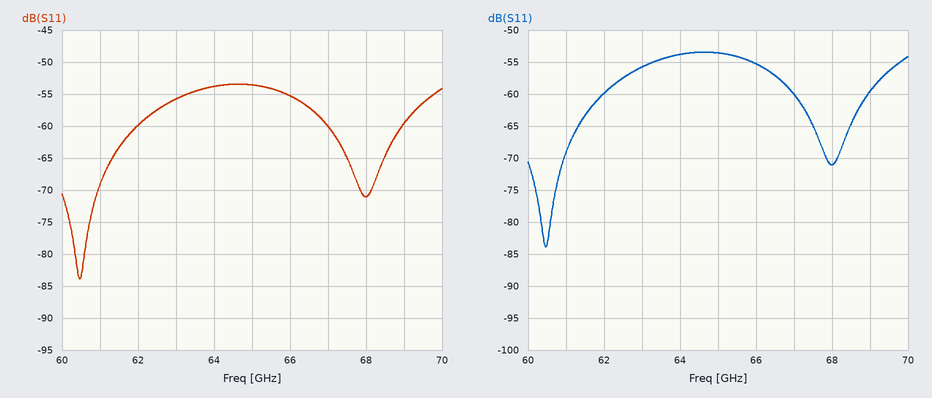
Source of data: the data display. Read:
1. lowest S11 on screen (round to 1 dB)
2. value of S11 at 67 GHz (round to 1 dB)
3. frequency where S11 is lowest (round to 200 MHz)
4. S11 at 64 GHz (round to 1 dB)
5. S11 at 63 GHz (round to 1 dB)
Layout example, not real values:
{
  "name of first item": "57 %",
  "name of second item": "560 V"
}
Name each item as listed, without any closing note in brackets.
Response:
{
  "lowest S11 on screen": "-84 dB",
  "value of S11 at 67 GHz": "-60 dB",
  "frequency where S11 is lowest": "60.4 GHz",
  "S11 at 64 GHz": "-54 dB",
  "S11 at 63 GHz": "-56 dB"
}
